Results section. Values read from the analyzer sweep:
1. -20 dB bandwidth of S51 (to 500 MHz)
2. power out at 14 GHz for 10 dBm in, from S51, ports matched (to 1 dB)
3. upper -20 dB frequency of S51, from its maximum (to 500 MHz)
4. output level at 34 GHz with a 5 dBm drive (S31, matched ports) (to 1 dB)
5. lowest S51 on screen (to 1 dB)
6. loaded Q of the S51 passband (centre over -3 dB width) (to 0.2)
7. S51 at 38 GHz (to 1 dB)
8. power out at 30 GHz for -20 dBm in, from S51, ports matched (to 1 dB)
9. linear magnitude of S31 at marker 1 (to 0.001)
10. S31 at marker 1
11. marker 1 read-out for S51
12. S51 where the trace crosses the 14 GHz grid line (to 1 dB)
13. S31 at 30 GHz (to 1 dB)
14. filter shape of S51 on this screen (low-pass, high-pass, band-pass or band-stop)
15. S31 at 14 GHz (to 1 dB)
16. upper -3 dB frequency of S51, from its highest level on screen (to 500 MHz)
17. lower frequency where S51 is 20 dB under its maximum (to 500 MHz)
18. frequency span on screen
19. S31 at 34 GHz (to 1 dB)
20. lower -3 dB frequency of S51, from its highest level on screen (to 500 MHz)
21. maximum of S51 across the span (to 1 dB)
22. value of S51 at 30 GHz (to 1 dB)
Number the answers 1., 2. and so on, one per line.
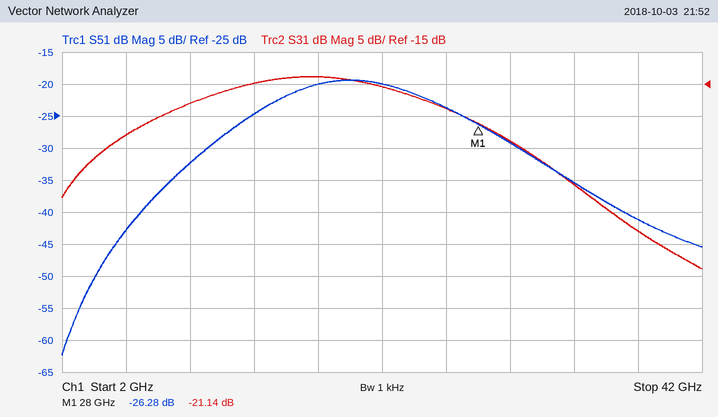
1. 29.5 GHz
2. -15 dBm
3. 36.5 GHz
4. -26 dBm
5. -62 dB
6. 2.2
7. -41 dB
8. -49 dBm
9. 0.088
10. -21.14 dB
11. -26.28 dB
12. -25 dB
13. -24 dB
14. band-pass
15. -15 dB
16. 25.0 GHz
17. 7.0 GHz
18. 40 GHz
19. -31 dB
20. 15.5 GHz
21. -19 dB
22. -29 dB
